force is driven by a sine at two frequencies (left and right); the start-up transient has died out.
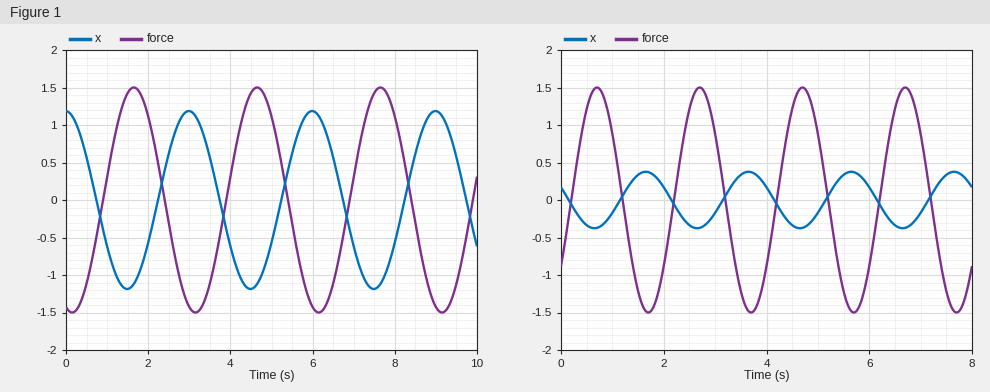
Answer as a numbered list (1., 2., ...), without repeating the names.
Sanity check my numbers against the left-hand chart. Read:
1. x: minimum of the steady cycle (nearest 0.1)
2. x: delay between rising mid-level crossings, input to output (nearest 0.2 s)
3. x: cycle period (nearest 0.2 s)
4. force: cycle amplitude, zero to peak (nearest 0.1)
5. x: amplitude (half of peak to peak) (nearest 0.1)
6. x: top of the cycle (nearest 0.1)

1. -1.2
2. 1.4 s
3. 3.0 s
4. 1.5
5. 1.2
6. 1.2
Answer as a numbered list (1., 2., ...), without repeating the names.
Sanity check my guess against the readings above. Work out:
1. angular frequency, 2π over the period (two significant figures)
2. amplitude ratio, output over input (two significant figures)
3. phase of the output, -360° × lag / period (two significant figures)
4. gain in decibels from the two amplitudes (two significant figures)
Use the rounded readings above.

1. 2.1 rad/s
2. 0.80
3. -170°
4. -1.9 dB
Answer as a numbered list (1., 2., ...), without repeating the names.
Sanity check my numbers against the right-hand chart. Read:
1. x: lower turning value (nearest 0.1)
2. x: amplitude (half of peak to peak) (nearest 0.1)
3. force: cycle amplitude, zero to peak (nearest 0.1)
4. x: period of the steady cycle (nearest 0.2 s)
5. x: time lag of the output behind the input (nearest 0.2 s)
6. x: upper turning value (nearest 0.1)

1. -0.4
2. 0.4
3. 1.5
4. 2.0 s
5. 1.0 s
6. 0.4
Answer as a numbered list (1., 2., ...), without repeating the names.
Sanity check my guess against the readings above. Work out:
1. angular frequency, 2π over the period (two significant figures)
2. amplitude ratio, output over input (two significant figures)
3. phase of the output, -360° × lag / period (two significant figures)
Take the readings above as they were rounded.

1. 3.1 rad/s
2. 0.27
3. -180°
